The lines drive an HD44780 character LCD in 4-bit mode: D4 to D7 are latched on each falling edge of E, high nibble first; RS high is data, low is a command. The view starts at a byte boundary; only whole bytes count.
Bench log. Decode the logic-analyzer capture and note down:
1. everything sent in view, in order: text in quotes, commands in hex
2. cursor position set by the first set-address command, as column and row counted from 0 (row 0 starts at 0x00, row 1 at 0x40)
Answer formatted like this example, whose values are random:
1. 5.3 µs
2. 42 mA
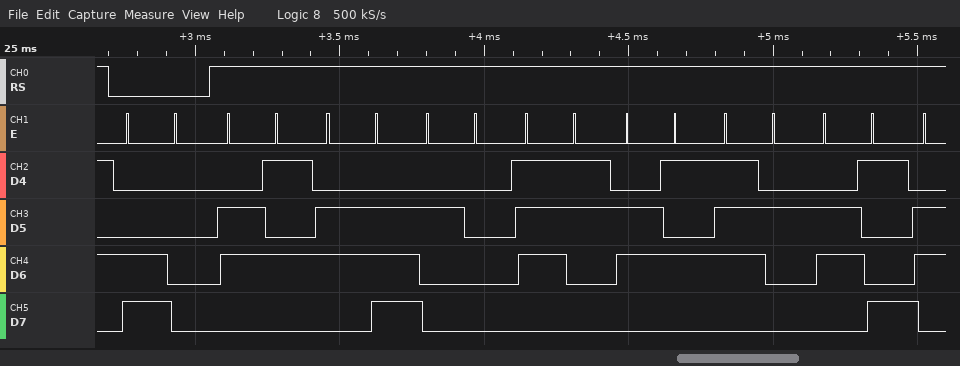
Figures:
1. 0xC0 "en seri"
2. column 0, row 1
